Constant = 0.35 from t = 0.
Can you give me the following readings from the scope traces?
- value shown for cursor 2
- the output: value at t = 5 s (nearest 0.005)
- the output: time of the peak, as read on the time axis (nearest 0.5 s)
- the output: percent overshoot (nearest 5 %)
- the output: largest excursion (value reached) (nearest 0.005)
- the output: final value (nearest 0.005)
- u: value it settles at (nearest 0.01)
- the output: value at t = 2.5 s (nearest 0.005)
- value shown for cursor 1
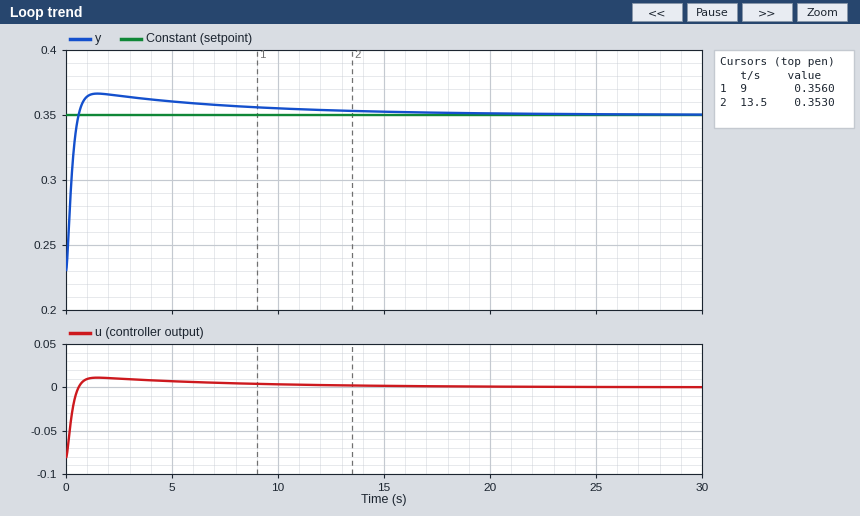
0.3530
0.360
1.5 s
15 %
0.365
0.350
0.00
0.365
0.3560
